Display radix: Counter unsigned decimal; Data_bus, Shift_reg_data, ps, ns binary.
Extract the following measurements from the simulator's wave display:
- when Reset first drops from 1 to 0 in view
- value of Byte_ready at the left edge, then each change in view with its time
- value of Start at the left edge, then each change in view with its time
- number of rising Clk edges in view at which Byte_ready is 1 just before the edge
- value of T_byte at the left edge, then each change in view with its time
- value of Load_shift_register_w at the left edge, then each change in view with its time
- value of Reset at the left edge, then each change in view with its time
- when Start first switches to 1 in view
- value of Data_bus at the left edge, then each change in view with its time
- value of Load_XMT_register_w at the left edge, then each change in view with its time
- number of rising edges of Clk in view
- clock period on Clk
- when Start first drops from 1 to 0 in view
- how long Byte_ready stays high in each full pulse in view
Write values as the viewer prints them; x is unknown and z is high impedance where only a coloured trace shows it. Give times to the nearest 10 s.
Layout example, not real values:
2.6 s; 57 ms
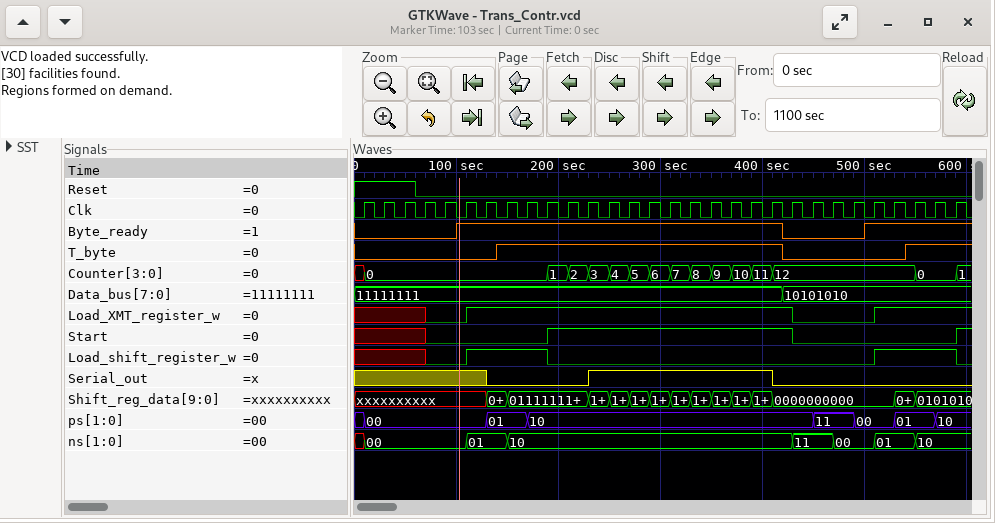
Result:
60 s; 0, 1 at 100 s, 0 at 420 s, 1 at 500 s; x, 0 at 70 s, 1 at 190 s, 0 at 430 s, 1 at 590 s; 21; 0, 1 at 140 s, 0 at 420 s, 1 at 540 s; x, 0 at 70 s, 1 at 110 s, 0 at 190 s, 1 at 510 s, 0 at 590 s; 1, 0 at 60 s; 190 s; 11111111, 10101010 at 420 s; x, 0 at 70 s, 1 at 110 s, 0 at 430 s, 1 at 510 s; 30; 20 s; 430 s; 320 s
